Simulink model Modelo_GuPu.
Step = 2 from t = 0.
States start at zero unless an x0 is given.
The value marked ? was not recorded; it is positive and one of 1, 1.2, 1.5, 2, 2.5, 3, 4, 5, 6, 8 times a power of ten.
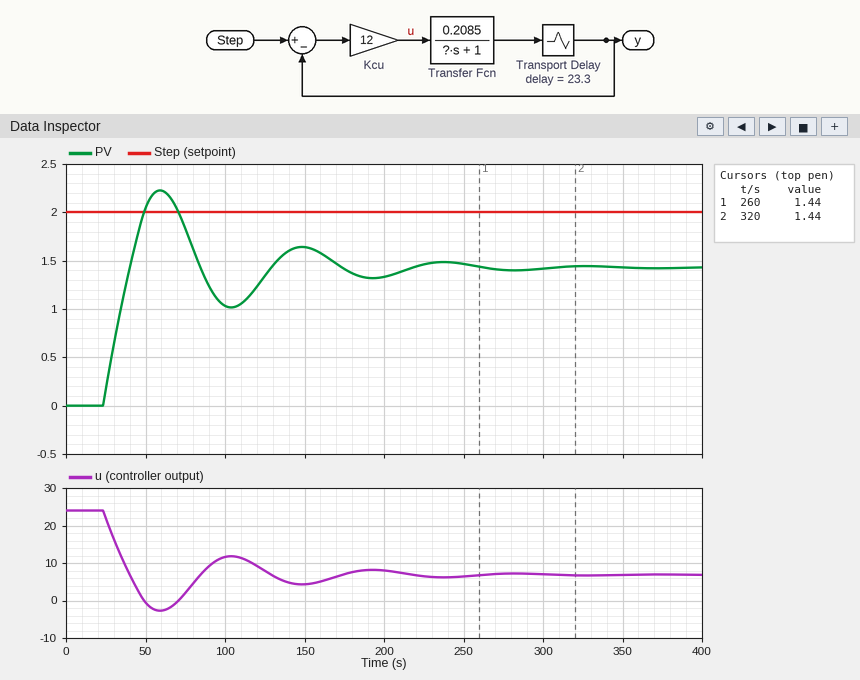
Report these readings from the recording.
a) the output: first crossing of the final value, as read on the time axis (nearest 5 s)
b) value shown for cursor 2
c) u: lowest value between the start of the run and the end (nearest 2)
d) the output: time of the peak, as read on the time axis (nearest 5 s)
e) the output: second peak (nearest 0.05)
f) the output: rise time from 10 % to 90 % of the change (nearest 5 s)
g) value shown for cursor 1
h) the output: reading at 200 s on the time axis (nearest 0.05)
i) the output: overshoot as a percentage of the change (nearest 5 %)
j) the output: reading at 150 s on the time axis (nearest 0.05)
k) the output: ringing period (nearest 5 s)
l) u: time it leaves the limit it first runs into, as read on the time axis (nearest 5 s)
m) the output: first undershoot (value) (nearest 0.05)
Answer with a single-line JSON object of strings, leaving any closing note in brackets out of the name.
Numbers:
{"the output: first crossing of the final value, as read on the time axis": "40 s", "value shown for cursor 2": "1.44", "u: lowest value between the start of the run and the end": "-2", "the output: time of the peak, as read on the time axis": "60 s", "the output: second peak": "1.65", "the output: rise time from 10 % to 90 % of the change": "15 s", "value shown for cursor 1": "1.44", "the output: reading at 200 s on the time axis": "1.35", "the output: overshoot as a percentage of the change": "55 %", "the output: reading at 150 s on the time axis": "1.65", "the output: ringing period": "90 s", "u: time it leaves the limit it first runs into, as read on the time axis": "25 s", "the output: first undershoot (value)": "1.00"}
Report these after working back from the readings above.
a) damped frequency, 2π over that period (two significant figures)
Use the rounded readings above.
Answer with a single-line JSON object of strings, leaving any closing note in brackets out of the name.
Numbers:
{"damped frequency, 2π over that period": "0.070 rad/s"}
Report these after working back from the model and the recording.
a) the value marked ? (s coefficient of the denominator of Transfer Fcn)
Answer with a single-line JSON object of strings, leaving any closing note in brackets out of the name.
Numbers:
{"the value marked ?": "50"}
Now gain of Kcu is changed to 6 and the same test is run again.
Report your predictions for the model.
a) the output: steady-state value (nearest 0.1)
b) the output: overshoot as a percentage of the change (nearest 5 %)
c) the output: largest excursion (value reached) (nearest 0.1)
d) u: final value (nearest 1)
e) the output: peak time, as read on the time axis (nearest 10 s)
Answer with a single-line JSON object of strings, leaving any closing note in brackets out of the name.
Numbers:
{"the output: steady-state value": "1.1", "the output: overshoot as a percentage of the change": "15 %", "the output: largest excursion (value reached)": "1.3", "u: final value": "5", "the output: peak time, as read on the time axis": "70 s"}
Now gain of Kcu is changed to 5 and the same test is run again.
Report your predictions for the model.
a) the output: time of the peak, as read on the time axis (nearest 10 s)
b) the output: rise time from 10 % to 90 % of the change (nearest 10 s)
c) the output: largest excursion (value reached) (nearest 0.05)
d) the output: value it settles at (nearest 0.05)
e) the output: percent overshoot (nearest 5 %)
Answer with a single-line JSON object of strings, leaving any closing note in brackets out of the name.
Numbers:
{"the output: time of the peak, as read on the time axis": "80 s", "the output: rise time from 10 % to 90 % of the change": "30 s", "the output: largest excursion (value reached)": "1.10", "the output: value it settles at": "1.00", "the output: percent overshoot": "10 %"}
